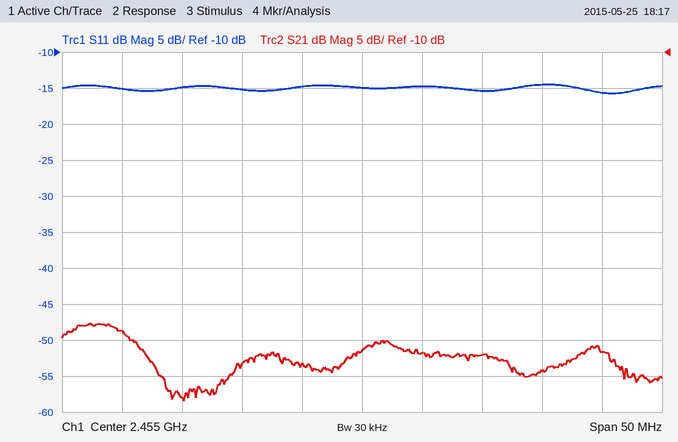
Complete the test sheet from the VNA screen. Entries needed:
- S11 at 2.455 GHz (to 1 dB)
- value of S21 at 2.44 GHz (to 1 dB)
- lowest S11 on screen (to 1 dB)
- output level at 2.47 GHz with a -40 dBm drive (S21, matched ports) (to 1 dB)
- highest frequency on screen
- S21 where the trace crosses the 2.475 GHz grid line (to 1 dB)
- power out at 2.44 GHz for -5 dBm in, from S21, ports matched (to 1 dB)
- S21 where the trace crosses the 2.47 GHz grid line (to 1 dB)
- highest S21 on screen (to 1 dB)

-15 dB
-58 dB
-16 dB
-94 dBm
2.48 GHz
-52 dB
-63 dBm
-54 dB
-48 dB
